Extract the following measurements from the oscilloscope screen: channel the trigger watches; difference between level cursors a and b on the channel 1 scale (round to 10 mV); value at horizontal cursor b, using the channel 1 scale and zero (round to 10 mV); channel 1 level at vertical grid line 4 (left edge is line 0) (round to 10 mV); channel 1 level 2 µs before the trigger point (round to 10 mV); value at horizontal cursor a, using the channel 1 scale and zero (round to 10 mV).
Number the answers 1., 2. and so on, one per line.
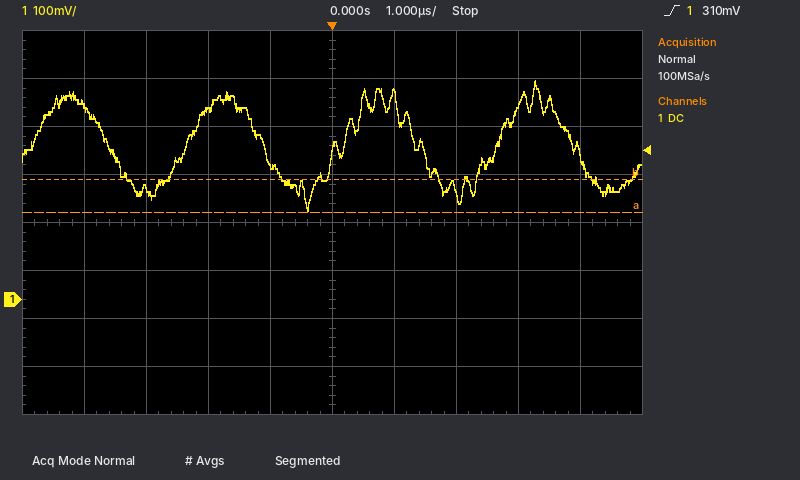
1. channel 1
2. 70 mV
3. 250 mV
4. 280 mV
5. 400 mV
6. 180 mV
